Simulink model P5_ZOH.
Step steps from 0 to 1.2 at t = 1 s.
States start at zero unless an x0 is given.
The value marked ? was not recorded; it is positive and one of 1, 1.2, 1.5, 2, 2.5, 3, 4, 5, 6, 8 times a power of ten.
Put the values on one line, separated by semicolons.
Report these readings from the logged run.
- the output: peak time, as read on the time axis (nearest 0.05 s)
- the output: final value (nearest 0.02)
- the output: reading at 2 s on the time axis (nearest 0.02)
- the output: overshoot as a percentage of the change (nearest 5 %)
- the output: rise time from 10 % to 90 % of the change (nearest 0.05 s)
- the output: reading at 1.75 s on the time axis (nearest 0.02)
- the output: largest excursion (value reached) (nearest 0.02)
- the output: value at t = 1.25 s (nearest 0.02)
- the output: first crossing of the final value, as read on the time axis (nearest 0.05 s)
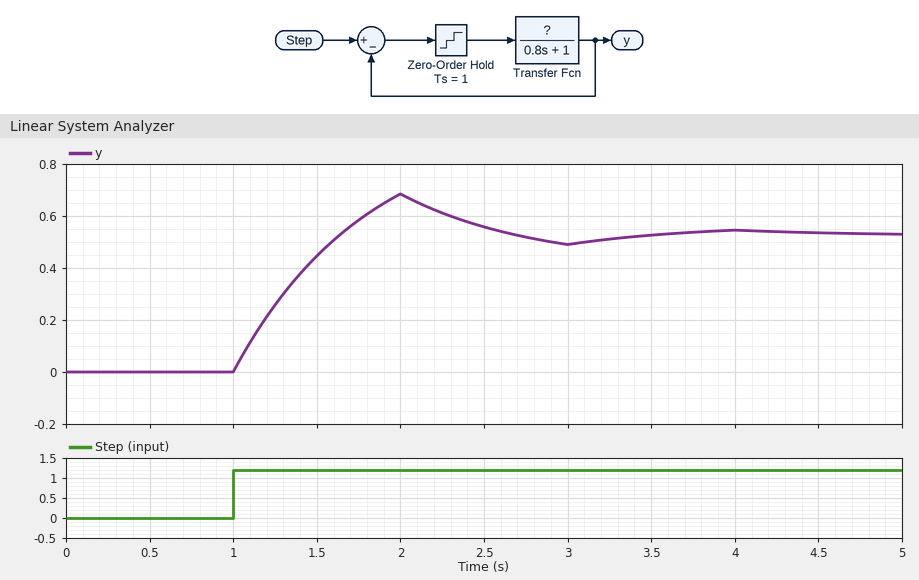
2.00 s; 0.54; 0.68; 30 %; 0.50 s; 0.58; 0.68; 0.26; 1.65 s
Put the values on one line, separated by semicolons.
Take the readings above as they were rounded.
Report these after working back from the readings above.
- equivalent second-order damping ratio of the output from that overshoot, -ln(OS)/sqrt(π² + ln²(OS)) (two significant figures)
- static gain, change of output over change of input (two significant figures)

0.36; 0.45
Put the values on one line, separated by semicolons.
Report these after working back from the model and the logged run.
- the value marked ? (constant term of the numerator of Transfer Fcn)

0.8
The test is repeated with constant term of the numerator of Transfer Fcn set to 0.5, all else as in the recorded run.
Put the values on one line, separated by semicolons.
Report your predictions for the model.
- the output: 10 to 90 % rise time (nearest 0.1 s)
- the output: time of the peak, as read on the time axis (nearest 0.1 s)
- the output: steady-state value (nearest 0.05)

0.7 s; 2.0 s; 0.40
